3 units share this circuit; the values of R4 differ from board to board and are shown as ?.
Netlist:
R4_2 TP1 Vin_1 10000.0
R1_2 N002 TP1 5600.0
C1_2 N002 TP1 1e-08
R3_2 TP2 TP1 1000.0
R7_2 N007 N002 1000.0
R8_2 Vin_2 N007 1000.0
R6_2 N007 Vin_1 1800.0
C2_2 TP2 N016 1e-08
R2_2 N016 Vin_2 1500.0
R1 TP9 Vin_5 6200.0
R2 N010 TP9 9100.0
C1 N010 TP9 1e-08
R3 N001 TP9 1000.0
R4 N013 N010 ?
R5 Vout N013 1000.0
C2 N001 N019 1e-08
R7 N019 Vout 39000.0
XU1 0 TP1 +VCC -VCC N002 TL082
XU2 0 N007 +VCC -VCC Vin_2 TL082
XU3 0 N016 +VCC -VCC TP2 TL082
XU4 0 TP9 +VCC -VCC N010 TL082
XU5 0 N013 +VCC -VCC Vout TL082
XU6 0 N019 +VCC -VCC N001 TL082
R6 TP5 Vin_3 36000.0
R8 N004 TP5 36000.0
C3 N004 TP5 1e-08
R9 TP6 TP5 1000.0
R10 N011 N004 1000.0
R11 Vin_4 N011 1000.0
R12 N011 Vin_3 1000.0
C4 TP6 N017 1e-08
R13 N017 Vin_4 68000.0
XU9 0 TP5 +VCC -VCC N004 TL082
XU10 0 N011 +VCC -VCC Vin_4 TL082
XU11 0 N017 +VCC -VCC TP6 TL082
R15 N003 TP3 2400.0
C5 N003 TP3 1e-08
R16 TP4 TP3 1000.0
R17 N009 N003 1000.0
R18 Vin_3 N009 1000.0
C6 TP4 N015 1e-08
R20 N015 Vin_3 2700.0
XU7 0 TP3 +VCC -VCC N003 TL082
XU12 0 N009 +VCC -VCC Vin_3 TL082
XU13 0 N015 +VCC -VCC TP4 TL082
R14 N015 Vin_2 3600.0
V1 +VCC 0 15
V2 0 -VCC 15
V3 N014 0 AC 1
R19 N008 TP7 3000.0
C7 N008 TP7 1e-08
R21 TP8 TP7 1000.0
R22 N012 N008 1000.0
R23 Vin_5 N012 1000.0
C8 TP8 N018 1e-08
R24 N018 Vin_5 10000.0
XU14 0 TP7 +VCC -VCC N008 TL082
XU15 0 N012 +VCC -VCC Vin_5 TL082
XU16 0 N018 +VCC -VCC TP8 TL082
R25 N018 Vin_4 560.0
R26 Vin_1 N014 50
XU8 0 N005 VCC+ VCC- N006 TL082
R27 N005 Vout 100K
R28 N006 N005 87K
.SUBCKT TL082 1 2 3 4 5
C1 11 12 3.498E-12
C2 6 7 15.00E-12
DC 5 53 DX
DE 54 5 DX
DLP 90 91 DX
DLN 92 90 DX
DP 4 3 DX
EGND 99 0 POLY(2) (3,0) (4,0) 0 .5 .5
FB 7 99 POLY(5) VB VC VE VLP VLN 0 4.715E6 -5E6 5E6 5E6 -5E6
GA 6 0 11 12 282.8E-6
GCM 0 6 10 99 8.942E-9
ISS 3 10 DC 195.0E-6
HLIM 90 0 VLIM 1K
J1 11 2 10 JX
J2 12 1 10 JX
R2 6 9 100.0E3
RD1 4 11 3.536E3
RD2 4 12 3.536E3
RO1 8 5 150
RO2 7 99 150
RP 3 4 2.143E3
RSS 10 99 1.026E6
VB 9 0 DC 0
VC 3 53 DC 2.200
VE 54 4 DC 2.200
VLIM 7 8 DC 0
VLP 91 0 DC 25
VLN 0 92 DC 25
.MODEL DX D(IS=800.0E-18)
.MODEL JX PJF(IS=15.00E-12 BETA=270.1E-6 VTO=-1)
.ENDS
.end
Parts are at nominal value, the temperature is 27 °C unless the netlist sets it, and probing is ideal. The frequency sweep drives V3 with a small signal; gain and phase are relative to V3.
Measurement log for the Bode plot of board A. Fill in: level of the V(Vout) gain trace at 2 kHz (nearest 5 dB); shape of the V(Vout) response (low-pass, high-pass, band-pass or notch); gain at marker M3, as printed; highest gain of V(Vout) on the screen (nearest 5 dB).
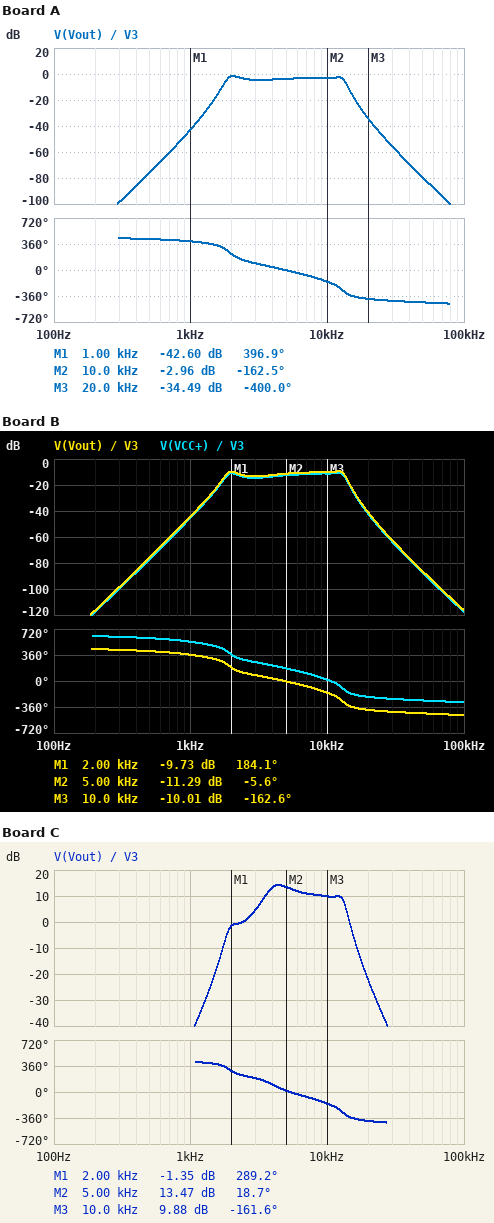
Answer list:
0 dB
band-pass
-34.49 dB
0 dB
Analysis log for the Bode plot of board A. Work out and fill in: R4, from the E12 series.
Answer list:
1.5 kΩ
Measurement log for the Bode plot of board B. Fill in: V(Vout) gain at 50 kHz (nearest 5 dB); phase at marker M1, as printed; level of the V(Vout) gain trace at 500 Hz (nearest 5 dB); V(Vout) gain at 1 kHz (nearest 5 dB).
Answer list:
-85 dB
184.1 deg
-75 dB
-45 dB
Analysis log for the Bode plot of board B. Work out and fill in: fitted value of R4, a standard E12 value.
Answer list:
3.3 kΩ
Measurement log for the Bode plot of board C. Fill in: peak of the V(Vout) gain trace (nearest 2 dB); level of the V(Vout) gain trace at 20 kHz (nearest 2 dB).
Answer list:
14 dB
-22 dB
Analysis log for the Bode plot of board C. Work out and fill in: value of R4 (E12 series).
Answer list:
390 Ω
